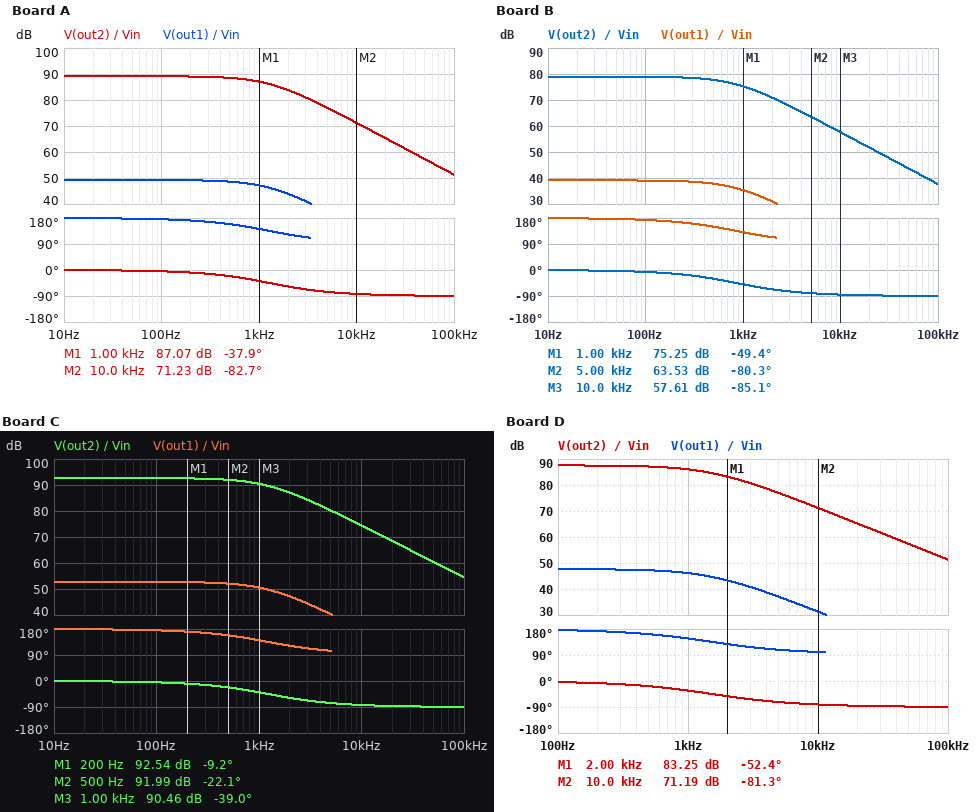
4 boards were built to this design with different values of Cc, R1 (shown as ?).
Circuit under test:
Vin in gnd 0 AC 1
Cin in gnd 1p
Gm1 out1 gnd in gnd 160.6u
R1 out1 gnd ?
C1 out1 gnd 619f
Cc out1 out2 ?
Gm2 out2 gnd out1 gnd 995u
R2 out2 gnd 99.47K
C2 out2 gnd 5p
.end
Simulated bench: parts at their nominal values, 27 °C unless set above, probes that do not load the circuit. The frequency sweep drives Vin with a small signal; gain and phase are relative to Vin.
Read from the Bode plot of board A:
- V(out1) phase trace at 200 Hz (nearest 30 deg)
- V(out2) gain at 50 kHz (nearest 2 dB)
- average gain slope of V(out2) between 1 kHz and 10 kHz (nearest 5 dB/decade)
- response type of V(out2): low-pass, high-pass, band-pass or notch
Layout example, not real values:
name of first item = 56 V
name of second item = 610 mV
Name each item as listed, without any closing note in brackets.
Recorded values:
V(out1) phase trace at 200 Hz = 180 deg
V(out2) gain at 50 kHz = 58 dB
average gain slope of V(out2) between 1 kHz and 10 kHz = -15 dB/decade
response type of V(out2): low-pass, high-pass, band-pass or notch = low-pass
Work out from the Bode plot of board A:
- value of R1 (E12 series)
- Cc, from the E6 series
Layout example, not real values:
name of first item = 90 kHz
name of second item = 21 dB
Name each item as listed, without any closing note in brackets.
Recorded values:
value of R1 = 1.8 MΩ
Cc, from the E6 series = 680 fF
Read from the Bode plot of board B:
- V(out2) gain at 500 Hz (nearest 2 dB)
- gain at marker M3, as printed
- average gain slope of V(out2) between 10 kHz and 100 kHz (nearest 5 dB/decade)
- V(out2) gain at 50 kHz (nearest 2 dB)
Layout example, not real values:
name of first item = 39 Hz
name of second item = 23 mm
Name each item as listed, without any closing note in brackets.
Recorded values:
V(out2) gain at 500 Hz = 78 dB
gain at marker M3, as printed = 57.61 dB
average gain slope of V(out2) between 10 kHz and 100 kHz = -20 dB/decade
V(out2) gain at 50 kHz = 44 dB
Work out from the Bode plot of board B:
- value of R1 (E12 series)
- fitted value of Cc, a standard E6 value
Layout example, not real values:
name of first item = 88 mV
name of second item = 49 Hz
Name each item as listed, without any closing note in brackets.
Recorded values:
value of R1 = 560 kΩ
fitted value of Cc, a standard E6 value = 3.3 pF
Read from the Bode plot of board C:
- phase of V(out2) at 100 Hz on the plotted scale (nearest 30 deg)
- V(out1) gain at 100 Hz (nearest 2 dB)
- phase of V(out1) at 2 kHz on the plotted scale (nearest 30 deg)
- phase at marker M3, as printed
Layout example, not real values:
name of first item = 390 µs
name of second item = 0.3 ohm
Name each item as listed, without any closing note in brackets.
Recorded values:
phase of V(out2) at 100 Hz on the plotted scale = 0 deg
V(out1) gain at 100 Hz = 52 dB
phase of V(out1) at 2 kHz on the plotted scale = 120 deg
phase at marker M3, as printed = -39.0 deg
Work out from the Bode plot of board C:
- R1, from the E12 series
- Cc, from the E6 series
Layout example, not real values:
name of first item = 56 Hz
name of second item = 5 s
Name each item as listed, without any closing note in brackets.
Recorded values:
R1, from the E12 series = 2.7 MΩ
Cc, from the E6 series = 470 fF
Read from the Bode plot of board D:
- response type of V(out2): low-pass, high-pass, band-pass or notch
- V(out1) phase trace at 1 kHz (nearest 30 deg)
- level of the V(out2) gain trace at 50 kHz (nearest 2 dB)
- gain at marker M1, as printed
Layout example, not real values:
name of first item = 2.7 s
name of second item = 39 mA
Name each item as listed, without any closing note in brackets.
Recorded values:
response type of V(out2): low-pass, high-pass, band-pass or notch = low-pass
V(out1) phase trace at 1 kHz = 150 deg
level of the V(out2) gain trace at 50 kHz = 58 dB
gain at marker M1, as printed = 83.25 dB
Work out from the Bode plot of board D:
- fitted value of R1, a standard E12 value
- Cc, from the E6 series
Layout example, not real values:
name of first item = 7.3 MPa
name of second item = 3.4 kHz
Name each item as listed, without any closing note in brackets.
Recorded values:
fitted value of R1, a standard E12 value = 1.5 MΩ
Cc, from the E6 series = 680 fF
